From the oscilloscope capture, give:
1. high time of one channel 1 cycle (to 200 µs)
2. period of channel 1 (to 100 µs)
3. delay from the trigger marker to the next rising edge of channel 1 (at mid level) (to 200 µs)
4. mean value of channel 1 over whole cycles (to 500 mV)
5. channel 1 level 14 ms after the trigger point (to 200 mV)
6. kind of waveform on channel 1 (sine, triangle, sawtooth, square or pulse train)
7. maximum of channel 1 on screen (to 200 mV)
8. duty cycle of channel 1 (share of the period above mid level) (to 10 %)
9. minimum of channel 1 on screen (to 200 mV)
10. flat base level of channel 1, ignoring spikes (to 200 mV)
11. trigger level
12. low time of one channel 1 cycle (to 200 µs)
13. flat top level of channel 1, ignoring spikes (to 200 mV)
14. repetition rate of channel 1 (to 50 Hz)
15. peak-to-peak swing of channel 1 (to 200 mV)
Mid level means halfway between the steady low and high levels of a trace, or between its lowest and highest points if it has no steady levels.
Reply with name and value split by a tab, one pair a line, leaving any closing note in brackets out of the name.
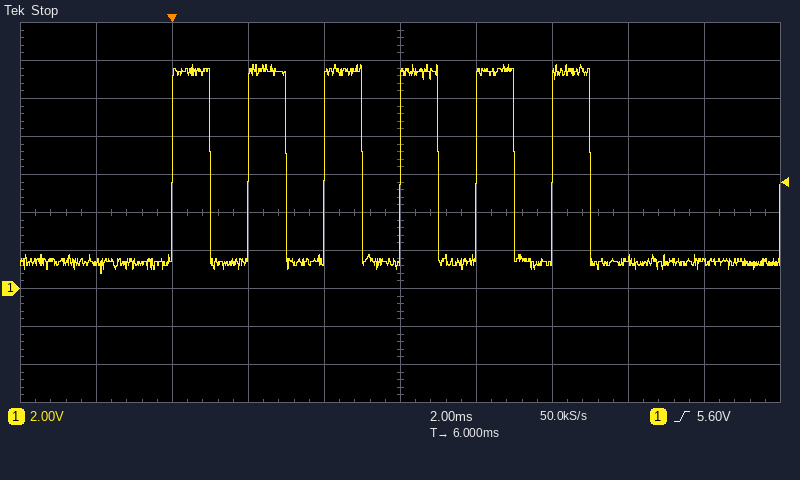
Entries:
high time of one channel 1 cycle	1.0 ms
period of channel 1	2.0 ms
delay from the trigger marker to the next rising edge of channel 1 (at mid level)	2.0 ms
mean value of channel 1 over whole cycles	6.5 V
channel 1 level 14 ms after the trigger point	1.4 V
kind of waveform on channel 1	square
maximum of channel 1 on screen	11.8 V
duty cycle of channel 1 (share of the period above mid level)	50 %
minimum of channel 1 on screen	800 mV
flat base level of channel 1, ignoring spikes	1.4 V
trigger level	5.60 V
low time of one channel 1 cycle	1.0 ms
flat top level of channel 1, ignoring spikes	11.4 V
repetition rate of channel 1	500 Hz
peak-to-peak swing of channel 1	11.0 V
